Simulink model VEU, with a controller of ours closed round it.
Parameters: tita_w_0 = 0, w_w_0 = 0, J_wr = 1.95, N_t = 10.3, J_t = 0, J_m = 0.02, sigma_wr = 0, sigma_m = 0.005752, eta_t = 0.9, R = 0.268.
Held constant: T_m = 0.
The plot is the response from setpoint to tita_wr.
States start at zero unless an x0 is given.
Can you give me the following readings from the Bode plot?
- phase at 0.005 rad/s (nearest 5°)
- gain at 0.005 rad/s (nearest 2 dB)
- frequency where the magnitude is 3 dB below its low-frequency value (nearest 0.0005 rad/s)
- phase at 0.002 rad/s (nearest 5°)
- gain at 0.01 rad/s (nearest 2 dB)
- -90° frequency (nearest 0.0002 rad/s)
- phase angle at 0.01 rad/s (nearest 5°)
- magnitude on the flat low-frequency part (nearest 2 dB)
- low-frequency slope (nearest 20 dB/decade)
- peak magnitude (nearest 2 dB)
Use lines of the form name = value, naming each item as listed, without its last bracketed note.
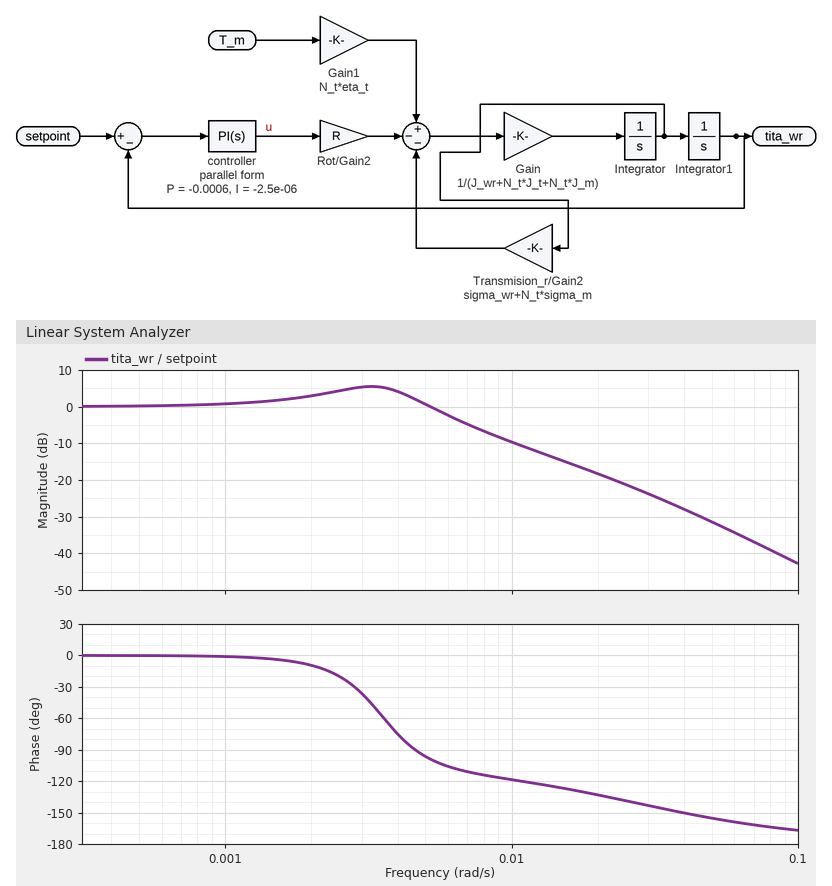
phase at 0.005 rad/s = -95°
gain at 0.005 rad/s = 0 dB
frequency where the magnitude is 3 dB below its low-frequency value = 0.0060 rad/s
phase at 0.002 rad/s = -10°
gain at 0.01 rad/s = -10 dB
-90° frequency = 0.0046 rad/s
phase angle at 0.01 rad/s = -120°
magnitude on the flat low-frequency part = 0 dB
low-frequency slope = 0 dB/decade
peak magnitude = 6 dB
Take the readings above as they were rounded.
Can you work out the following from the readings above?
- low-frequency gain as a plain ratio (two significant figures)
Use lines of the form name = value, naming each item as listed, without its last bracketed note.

low-frequency gain as a plain ratio = 1.0
